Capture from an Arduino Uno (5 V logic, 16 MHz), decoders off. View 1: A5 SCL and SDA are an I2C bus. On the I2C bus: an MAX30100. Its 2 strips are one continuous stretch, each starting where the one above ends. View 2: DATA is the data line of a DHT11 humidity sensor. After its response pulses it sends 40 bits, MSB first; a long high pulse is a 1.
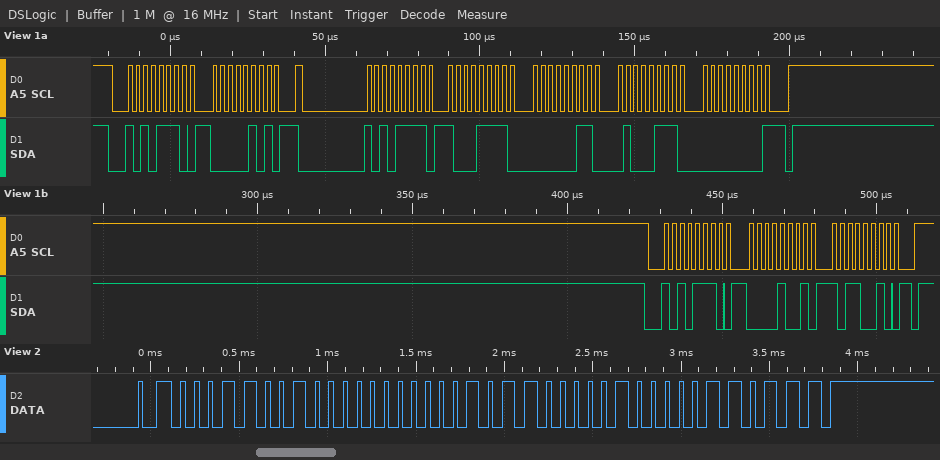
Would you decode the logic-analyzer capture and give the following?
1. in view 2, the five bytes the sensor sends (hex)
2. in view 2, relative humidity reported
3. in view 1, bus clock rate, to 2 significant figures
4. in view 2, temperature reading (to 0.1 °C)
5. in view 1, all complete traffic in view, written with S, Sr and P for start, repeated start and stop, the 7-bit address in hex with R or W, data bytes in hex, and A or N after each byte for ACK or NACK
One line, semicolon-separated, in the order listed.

19 00 16 08 37; 25 %; 400 kHz; 22.8 °C; S 57W A 05 A Sr 57R A 8F A 03 A 47 A 00 N P S 57W A 09 A B2 A P
